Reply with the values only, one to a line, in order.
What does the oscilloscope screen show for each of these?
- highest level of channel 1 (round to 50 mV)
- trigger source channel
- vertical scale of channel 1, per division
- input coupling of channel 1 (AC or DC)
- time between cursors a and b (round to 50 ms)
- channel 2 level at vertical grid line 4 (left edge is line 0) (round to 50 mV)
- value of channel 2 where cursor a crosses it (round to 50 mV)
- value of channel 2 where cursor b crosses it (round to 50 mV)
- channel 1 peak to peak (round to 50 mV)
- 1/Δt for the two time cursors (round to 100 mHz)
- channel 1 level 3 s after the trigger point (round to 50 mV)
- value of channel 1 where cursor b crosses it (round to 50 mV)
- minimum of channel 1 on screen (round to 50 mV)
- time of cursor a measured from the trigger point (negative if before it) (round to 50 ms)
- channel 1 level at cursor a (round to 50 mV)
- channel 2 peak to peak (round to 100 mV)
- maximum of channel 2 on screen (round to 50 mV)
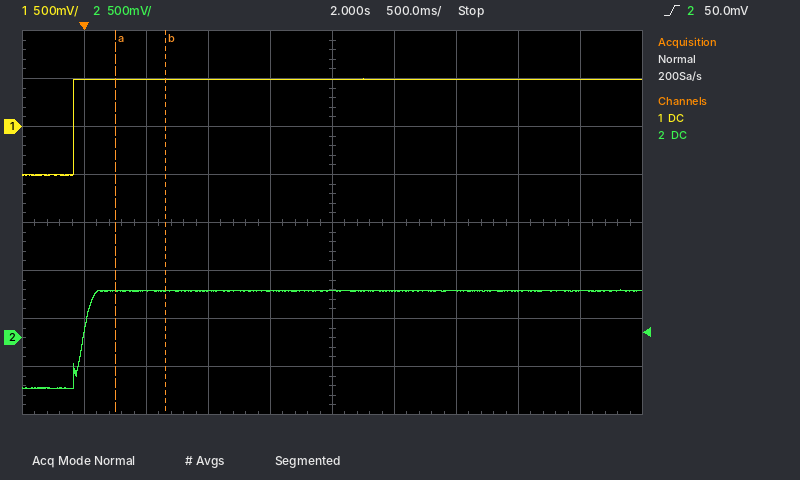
500 mV
channel 2
500 mV
DC
400 ms
500 mV
500 mV
500 mV
1.00 V
2.5 Hz
500 mV
500 mV
-500 mV
+250 ms
500 mV
1.00 V
500 mV
